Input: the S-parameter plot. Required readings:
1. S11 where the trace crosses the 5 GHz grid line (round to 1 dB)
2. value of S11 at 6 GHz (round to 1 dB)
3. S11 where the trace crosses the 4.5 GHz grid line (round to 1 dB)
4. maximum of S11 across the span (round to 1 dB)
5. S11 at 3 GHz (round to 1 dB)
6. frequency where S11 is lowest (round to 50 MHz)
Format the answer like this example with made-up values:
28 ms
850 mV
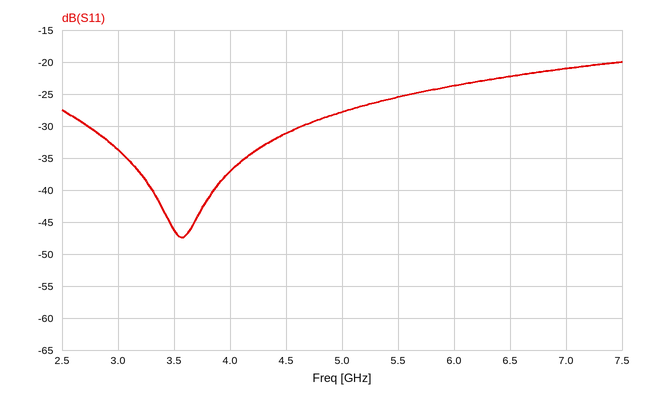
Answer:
-28 dB
-24 dB
-31 dB
-20 dB
-34 dB
3.55 GHz
